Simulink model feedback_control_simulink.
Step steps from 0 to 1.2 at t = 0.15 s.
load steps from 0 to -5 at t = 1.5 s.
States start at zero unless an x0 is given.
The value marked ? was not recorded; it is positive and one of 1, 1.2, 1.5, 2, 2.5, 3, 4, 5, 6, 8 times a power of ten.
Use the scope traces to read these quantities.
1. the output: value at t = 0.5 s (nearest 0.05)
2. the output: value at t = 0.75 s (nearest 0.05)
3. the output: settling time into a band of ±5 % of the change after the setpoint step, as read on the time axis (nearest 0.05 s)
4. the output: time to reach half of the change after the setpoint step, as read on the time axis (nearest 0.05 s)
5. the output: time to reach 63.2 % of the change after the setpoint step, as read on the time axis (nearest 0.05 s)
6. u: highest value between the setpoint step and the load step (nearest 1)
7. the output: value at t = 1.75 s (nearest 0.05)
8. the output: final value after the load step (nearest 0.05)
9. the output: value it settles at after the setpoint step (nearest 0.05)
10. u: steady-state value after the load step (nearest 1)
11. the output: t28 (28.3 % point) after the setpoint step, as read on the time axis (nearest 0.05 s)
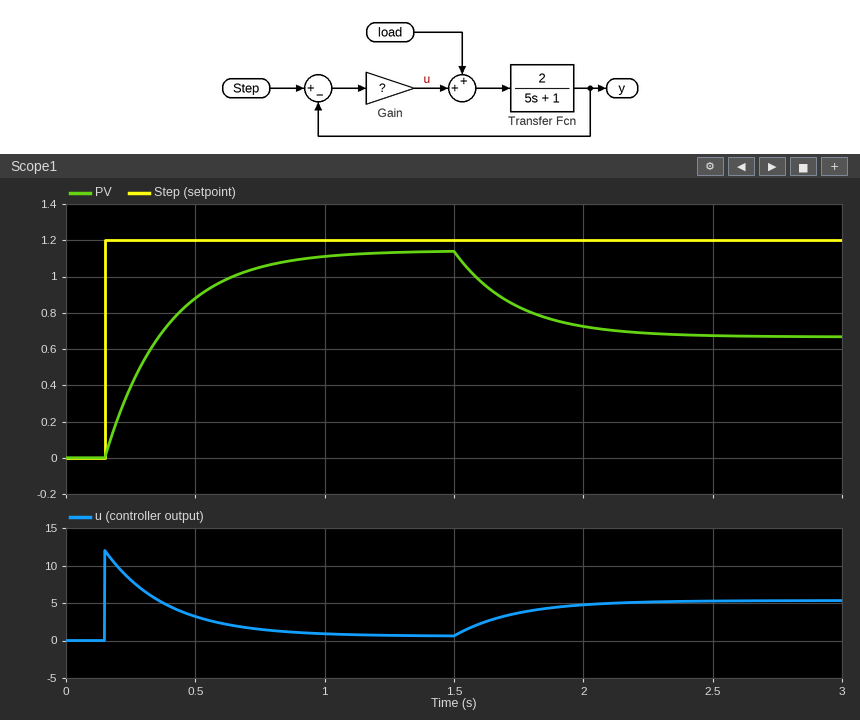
0.90
1.05
0.85 s
0.30 s
0.40 s
12
0.85
0.65
1.15
5
0.25 s
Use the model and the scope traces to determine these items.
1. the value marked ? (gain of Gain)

10
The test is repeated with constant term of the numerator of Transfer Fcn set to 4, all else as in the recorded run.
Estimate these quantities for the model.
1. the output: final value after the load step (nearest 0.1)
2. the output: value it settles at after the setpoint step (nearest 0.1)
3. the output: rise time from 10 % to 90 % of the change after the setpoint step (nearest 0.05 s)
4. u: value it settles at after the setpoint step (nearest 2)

0.7
1.2
0.25 s
0
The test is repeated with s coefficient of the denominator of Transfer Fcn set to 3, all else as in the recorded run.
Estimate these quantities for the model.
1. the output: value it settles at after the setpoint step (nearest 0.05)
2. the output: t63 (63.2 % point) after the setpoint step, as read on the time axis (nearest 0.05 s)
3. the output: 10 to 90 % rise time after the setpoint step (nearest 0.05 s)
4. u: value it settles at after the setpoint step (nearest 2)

1.15
0.30 s
0.30 s
0
